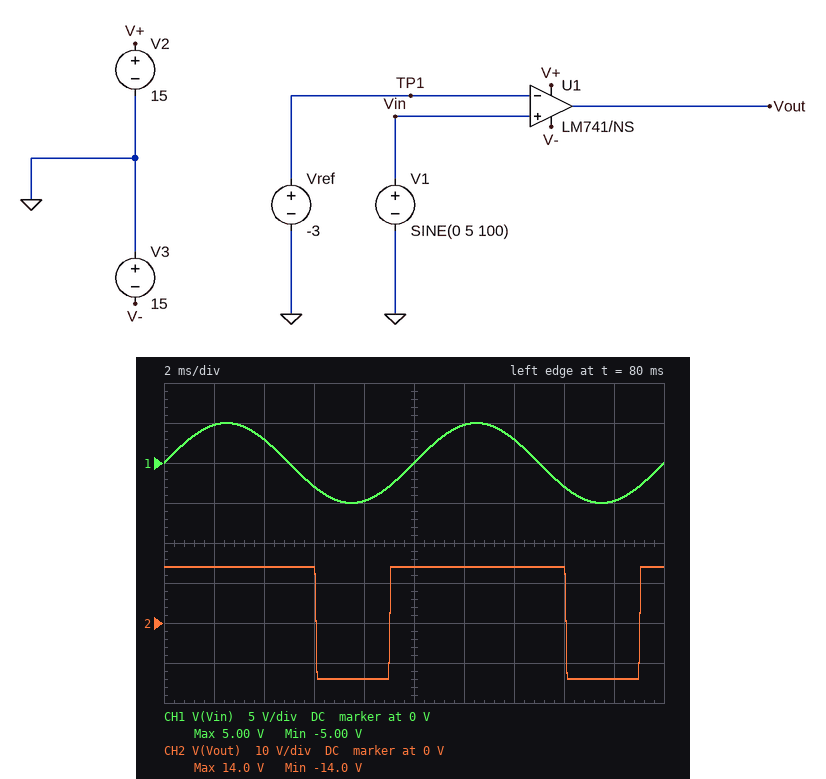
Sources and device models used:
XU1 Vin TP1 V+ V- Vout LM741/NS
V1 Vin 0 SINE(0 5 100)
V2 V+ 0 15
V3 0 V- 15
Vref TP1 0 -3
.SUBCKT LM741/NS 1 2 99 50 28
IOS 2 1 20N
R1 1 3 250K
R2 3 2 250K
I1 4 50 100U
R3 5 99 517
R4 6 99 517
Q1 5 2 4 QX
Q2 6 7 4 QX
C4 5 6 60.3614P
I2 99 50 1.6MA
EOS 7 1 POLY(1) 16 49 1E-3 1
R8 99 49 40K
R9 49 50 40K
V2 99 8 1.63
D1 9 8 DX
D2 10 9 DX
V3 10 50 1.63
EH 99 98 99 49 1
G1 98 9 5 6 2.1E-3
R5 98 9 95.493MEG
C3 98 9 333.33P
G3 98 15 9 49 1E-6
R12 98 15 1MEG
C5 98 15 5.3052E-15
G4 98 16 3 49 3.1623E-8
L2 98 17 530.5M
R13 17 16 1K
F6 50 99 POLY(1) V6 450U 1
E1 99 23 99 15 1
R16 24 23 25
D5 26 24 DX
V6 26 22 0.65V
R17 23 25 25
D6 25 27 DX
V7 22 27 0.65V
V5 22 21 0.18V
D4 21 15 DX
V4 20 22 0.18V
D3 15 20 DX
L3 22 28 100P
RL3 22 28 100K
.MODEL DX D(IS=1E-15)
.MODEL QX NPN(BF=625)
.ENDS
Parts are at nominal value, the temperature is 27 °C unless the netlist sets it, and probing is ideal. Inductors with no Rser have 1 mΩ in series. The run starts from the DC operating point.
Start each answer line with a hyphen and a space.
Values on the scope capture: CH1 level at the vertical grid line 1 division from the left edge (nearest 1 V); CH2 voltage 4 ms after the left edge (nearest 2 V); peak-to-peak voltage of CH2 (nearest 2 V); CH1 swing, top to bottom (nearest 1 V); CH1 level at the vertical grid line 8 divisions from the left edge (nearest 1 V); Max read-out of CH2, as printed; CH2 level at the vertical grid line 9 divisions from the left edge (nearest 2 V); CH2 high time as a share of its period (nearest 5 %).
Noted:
- 5 V
- 14 V
- 28 V
- 10 V
- -3 V
- 14.0 V
- -14 V
- 70 %
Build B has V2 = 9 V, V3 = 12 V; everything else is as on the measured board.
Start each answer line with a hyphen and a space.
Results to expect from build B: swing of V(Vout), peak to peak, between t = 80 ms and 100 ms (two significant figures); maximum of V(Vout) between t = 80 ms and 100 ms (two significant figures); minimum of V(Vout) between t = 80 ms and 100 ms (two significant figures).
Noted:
- 19 V
- 8.0 V
- -11 V
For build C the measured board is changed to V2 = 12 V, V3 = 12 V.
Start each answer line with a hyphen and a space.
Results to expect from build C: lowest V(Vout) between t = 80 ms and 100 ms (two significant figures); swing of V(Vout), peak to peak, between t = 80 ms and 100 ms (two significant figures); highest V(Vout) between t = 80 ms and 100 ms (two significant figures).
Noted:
- -11 V
- 22 V
- 11 V
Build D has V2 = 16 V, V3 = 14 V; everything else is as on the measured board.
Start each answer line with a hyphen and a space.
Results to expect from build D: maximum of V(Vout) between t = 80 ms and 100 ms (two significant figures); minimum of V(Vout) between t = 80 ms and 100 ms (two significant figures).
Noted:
- 15 V
- -13 V
